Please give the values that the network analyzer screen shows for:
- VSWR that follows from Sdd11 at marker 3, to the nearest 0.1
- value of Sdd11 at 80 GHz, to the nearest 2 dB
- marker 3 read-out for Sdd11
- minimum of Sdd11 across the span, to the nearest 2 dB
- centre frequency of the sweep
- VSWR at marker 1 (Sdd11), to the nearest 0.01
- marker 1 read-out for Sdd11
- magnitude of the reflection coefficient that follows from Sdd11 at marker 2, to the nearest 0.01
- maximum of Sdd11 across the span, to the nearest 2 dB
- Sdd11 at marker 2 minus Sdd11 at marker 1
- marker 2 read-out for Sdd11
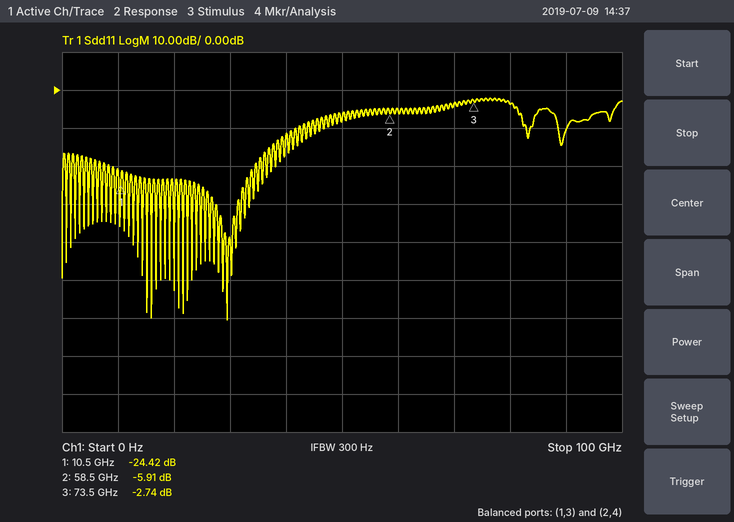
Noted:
6.4
-4 dB
-2.74 dB
-60 dB
50 GHz
1.13
-24.42 dB
0.51
-2 dB
18.51 dB
-5.91 dB
